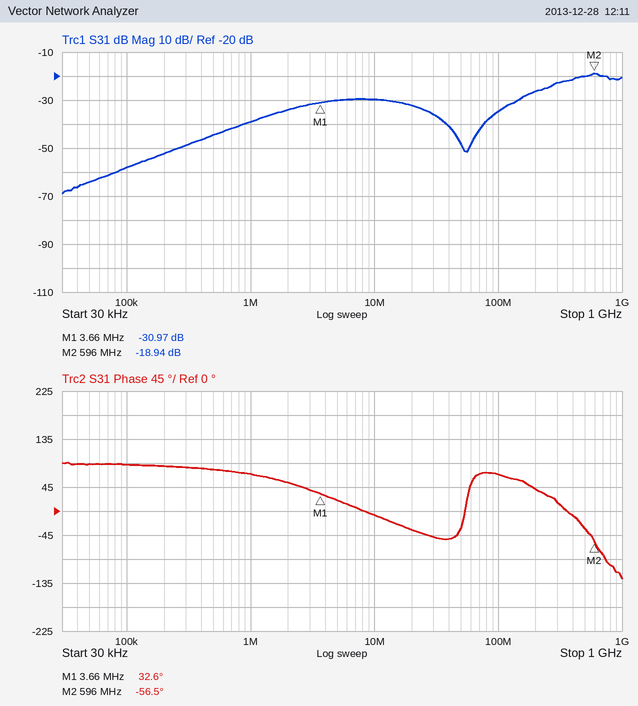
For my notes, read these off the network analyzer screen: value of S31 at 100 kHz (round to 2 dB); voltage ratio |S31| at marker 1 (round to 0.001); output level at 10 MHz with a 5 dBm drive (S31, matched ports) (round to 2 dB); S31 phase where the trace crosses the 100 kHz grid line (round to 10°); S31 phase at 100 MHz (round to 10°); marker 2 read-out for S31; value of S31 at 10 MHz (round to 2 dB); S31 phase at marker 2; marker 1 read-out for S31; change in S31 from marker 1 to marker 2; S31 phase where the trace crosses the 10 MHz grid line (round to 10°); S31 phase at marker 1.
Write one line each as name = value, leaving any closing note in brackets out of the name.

value of S31 at 100 kHz = -58 dB
voltage ratio |S31| at marker 1 = 0.028
output level at 10 MHz with a 5 dBm drive (S31, matched ports) = -24 dBm
S31 phase where the trace crosses the 100 kHz grid line = 90°
S31 phase at 100 MHz = 70°
marker 2 read-out for S31 = -18.94 dB
value of S31 at 10 MHz = -30 dB
S31 phase at marker 2 = -56.5°
marker 1 read-out for S31 = -30.97 dB
change in S31 from marker 1 to marker 2 = 12.03 dB
S31 phase where the trace crosses the 10 MHz grid line = -10°
S31 phase at marker 1 = 32.6°
